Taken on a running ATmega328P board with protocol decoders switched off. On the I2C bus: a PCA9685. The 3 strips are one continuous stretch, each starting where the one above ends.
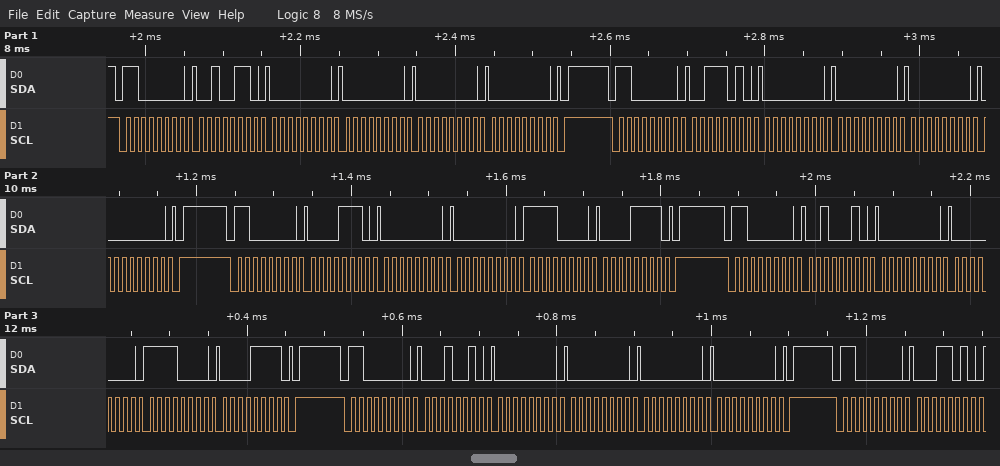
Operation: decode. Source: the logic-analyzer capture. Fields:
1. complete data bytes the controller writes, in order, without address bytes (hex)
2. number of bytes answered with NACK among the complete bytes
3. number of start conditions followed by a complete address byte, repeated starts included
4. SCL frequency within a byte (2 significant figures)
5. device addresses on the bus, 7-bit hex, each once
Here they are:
26 00 00 00 00 3A 00 00 00 00 0E 00 00 F0 0F 22 00 00 F0 0F 12 00 00 00 00 1A
0
6
100 kHz
0x60
